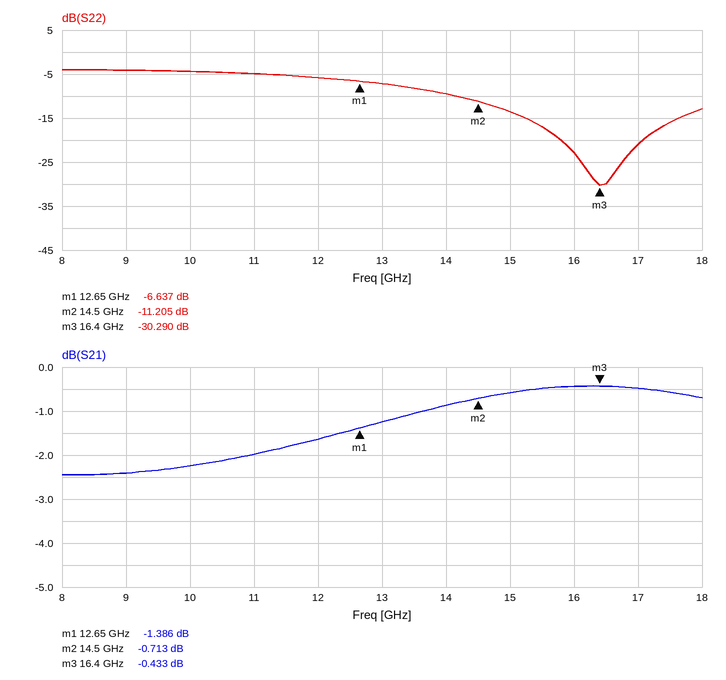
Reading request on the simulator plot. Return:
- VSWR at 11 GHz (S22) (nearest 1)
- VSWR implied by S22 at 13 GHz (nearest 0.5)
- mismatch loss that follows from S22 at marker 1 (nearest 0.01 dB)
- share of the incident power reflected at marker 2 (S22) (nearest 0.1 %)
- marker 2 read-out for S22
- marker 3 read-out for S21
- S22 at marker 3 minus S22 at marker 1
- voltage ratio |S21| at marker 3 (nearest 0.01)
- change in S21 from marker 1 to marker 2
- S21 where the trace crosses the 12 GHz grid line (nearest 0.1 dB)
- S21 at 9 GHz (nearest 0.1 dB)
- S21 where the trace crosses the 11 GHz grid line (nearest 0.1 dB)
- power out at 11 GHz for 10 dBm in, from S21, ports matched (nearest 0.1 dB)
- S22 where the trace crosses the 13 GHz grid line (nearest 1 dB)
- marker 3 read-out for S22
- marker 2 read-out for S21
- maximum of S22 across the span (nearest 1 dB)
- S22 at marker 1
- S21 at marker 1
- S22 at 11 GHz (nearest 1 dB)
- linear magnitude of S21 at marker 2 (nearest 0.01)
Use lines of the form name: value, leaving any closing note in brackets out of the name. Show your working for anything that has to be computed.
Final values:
VSWR at 11 GHz (S22): |Γ| = 10^(-5/20) = 0.5623; VSWR = (1 + 0.5623)/(1 − 0.5623) ≈ 4
VSWR implied by S22 at 13 GHz: |Γ| = 10^(-7/20) = 0.4467; VSWR = (1 + 0.4467)/(1 − 0.4467) ≈ 2.61, so 2.5 to the nearest 0.5
mismatch loss that follows from S22 at marker 1: −10 log10(1 − 10^(-6.637/10)) ≈ 1.06 dB
share of the incident power reflected at marker 2 (S22): 10^(-11.205/10) ≈ 7.6 %
marker 2 read-out for S22: -11.205 dB
marker 3 read-out for S21: -0.433 dB
S22 at marker 3 minus S22 at marker 1: -30.29 − (-6.637) = -23.653 dB
voltage ratio |S21| at marker 3: 10^(-0.433/20) ≈ 0.95
change in S21 from marker 1 to marker 2: -0.713 − (-1.386) = 0.673 dB
S21 where the trace crosses the 12 GHz grid line: -1.6 dB
S21 at 9 GHz: -2.4 dB
S21 where the trace crosses the 11 GHz grid line: -2.0 dB
power out at 11 GHz for 10 dBm in, from S21, ports matched: 10 dBm + (-2.0 dB) = 8.0 dBm
S22 where the trace crosses the 13 GHz grid line: -7 dB
marker 3 read-out for S22: -30.290 dB
marker 2 read-out for S21: -0.713 dB
maximum of S22 across the span: -4 dB
S22 at marker 1: -6.637 dB
S21 at marker 1: -1.386 dB
S22 at 11 GHz: -5 dB
linear magnitude of S21 at marker 2: 10^(-0.713/20) ≈ 0.92
